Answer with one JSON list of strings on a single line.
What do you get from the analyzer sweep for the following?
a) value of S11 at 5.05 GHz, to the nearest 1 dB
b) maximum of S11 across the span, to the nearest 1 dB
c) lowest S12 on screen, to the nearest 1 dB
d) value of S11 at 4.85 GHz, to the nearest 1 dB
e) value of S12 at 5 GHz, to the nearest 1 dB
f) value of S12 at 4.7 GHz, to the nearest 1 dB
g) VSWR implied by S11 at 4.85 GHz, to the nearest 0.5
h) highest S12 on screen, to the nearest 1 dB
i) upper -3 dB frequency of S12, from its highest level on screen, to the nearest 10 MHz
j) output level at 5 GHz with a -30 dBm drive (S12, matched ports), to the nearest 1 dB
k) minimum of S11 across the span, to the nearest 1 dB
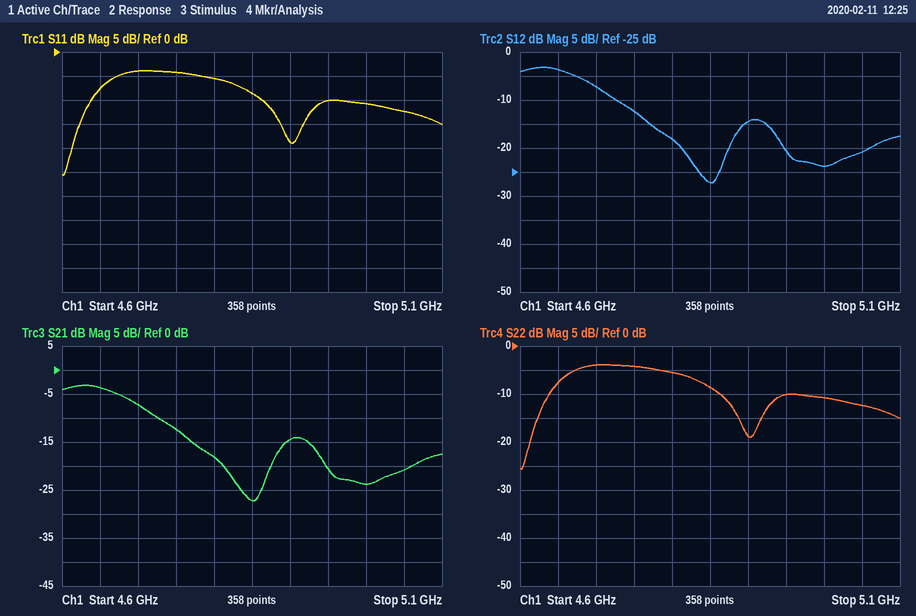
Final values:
["-12 dB", "-4 dB", "-27 dB", "-9 dB", "-24 dB", "-7 dB", "2.0", "-3 dB", "4.69 GHz", "-54 dBm", "-26 dB"]
